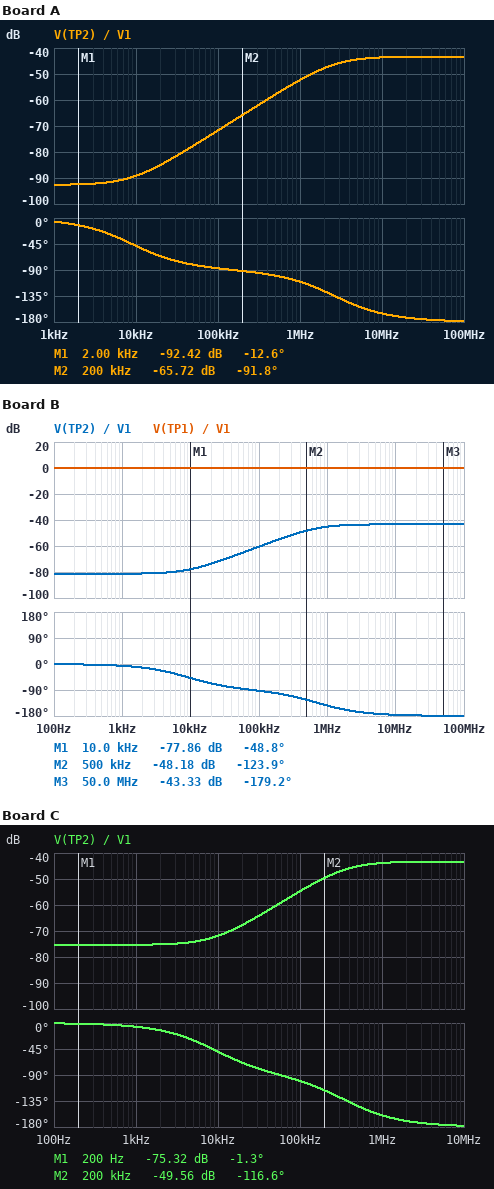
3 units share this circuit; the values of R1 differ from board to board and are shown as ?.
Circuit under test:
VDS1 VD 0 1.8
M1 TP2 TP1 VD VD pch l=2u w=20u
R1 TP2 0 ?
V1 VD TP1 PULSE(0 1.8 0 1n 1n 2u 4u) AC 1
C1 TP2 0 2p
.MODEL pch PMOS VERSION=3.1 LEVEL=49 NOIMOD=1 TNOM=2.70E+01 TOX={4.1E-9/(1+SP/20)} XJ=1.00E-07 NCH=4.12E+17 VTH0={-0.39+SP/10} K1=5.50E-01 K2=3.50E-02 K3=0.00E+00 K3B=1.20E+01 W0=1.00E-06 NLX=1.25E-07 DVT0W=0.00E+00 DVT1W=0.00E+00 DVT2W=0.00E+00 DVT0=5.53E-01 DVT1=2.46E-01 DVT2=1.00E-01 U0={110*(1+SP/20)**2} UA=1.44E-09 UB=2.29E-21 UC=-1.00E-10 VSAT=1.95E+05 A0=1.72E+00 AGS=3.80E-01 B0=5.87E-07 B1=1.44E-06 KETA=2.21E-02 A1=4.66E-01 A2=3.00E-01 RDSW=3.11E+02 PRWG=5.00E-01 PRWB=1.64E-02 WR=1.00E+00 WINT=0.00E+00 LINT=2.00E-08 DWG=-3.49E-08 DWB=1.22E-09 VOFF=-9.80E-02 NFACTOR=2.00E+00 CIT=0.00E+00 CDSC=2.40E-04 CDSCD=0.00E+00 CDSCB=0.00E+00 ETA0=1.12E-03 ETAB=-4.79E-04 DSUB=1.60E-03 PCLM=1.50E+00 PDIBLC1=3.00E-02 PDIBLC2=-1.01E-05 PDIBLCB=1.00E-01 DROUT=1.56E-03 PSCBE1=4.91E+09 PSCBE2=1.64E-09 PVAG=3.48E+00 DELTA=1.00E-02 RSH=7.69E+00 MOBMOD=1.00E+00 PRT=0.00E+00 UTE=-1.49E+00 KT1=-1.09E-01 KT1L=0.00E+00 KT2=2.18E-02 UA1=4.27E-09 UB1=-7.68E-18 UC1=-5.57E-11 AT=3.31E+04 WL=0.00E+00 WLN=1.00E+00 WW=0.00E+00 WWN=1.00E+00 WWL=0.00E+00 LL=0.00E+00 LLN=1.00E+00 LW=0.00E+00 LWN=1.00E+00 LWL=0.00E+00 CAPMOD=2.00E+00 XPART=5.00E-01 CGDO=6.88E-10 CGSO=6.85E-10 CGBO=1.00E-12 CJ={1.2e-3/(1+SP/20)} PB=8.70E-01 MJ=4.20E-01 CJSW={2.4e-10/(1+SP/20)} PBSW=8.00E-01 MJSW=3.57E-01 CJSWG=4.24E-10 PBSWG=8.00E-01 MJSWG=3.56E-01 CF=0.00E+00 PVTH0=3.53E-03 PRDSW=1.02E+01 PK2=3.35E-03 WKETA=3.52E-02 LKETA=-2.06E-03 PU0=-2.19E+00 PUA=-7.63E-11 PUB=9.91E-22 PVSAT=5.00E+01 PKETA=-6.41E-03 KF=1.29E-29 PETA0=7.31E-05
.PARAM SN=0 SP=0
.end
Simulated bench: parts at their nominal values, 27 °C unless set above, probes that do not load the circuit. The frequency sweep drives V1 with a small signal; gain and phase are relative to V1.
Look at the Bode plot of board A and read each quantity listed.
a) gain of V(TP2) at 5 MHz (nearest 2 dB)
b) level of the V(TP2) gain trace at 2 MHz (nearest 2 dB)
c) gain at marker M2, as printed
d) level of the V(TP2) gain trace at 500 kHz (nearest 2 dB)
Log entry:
-44 dB
-48 dB
-65.72 dB
-58 dB
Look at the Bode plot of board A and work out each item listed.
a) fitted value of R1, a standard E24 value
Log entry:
30 kΩ
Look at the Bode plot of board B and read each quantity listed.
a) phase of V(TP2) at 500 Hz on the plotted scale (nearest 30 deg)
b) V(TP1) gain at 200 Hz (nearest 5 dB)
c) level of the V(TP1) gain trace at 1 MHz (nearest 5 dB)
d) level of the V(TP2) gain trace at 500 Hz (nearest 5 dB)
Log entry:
0 deg
0 dB
0 dB
-80 dB
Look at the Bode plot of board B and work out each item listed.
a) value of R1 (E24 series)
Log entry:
110 kΩ
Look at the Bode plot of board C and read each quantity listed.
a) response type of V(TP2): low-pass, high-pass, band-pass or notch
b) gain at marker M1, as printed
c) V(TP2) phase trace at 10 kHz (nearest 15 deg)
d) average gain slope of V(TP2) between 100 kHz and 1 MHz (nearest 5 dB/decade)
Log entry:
high-pass
-75.32 dB
-45 deg
10 dB/decade
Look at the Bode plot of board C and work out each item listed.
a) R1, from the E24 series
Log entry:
220 kΩ
